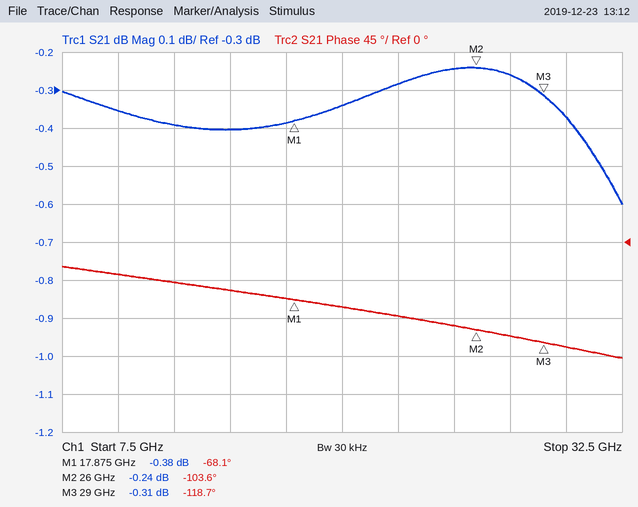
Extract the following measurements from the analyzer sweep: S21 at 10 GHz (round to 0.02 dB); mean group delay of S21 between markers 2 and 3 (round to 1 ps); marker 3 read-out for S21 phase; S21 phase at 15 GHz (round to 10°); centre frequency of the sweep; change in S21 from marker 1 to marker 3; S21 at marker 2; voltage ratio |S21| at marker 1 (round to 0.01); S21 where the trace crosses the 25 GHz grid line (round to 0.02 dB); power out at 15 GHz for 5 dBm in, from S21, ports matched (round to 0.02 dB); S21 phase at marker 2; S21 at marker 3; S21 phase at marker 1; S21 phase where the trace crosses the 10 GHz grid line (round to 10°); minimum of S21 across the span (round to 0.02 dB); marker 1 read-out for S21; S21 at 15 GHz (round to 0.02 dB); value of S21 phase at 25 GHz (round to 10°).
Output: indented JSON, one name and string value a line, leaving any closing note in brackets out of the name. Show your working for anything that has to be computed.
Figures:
{
  "S21 at 10 GHz": "-0.36 dB",
  "mean group delay of S21 between markers 2 and 3": "−(-118.7° − (-103.6°))/(360° × 3 GHz) ≈ 14 ps",
  "marker 3 read-out for S21 phase": "-118.7°",
  "S21 phase at 15 GHz": "-60°",
  "centre frequency of the sweep": "20 GHz",
  "change in S21 from marker 1 to marker 3": "-0.31 − (-0.38) = 0.07 dB",
  "S21 at marker 2": "-0.24 dB",
  "voltage ratio |S21| at marker 1": "10^(-0.38/20) ≈ 0.96",
  "S21 where the trace crosses the 25 GHz grid line": "-0.24 dB",
  "power out at 15 GHz for 5 dBm in, from S21, ports matched": "5 dBm + (-0.40 dB) = 4.60 dBm",
  "S21 phase at marker 2": "-103.6°",
  "S21 at marker 3": "-0.31 dB",
  "S21 phase at marker 1": "-68.1°",
  "S21 phase where the trace crosses the 10 GHz grid line": "-40°",
  "minimum of S21 across the span": "-0.60 dB",
  "marker 1 read-out for S21": "-0.38 dB",
  "S21 at 15 GHz": "-0.40 dB",
  "value of S21 phase at 25 GHz": "-100°"
}
